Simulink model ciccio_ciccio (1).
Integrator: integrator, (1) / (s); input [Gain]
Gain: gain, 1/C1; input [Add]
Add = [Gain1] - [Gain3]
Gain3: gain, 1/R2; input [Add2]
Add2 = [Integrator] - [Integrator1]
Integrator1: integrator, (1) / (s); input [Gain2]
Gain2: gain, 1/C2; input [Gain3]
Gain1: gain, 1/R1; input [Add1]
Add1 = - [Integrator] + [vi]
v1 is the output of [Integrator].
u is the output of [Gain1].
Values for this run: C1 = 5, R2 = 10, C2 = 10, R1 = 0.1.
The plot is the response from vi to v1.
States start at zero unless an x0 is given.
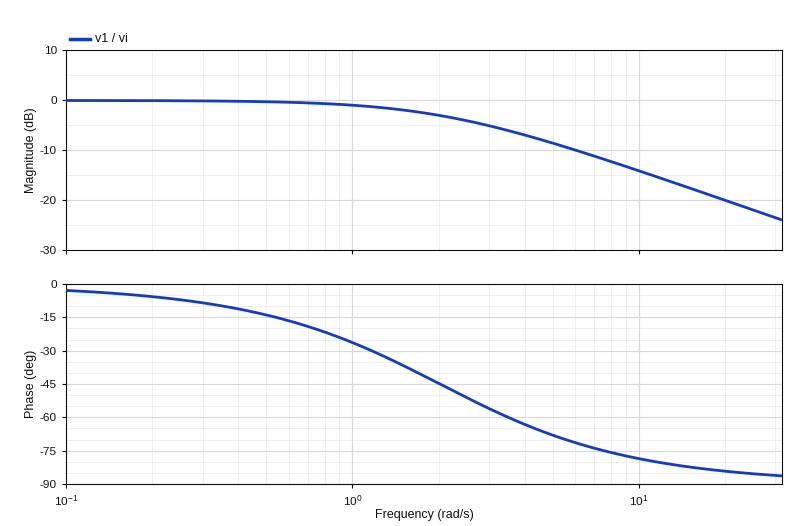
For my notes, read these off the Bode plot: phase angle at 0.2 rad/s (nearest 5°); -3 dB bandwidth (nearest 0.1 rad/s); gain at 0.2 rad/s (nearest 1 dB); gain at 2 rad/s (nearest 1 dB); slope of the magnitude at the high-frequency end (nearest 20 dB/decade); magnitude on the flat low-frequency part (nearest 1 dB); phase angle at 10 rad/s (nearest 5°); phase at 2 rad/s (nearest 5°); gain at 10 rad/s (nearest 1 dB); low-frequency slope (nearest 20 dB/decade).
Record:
-5°
2.0 rad/s
0 dB
-3 dB
-20 dB/decade
0 dB
-80°
-45°
-14 dB
0 dB/decade
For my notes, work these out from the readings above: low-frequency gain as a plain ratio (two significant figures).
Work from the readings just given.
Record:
1.0
